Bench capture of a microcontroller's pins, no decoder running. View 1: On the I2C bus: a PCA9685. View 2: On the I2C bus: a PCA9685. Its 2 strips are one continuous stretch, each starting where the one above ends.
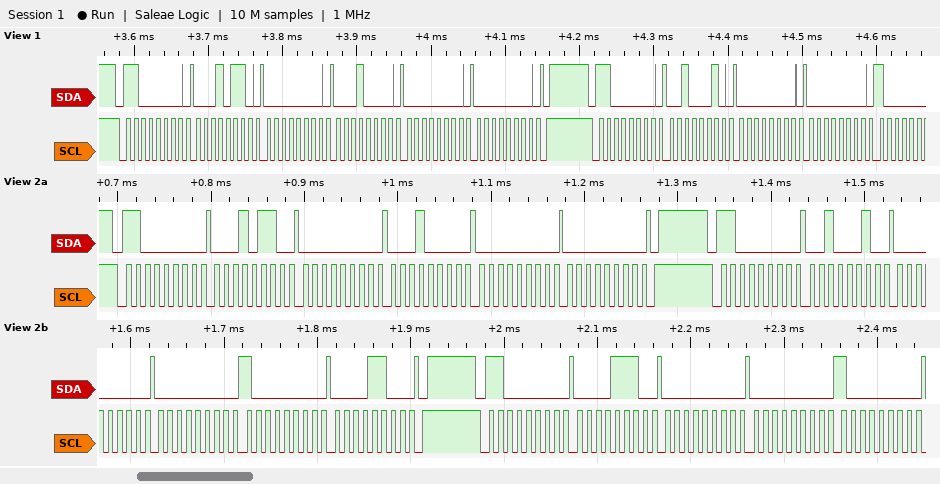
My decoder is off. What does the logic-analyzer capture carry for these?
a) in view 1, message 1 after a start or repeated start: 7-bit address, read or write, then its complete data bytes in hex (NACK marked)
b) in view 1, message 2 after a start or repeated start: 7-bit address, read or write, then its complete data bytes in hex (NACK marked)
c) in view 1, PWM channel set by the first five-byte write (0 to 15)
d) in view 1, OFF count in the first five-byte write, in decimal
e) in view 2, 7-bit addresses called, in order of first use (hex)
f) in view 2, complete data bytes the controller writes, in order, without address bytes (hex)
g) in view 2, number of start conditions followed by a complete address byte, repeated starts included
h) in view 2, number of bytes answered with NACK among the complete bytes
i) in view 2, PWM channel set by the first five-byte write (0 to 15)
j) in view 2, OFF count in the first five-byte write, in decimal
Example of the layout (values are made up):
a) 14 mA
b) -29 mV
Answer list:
a) 0x60 write: 16 00 10 00 00
b) 0x60 write: 22 00 00
c) 4
d) 0
e) 0x60
f) 16 00 10 00 00 22 00 00 80 0C 0E 00 00 80
g) 3
h) 0
i) 4
j) 0
